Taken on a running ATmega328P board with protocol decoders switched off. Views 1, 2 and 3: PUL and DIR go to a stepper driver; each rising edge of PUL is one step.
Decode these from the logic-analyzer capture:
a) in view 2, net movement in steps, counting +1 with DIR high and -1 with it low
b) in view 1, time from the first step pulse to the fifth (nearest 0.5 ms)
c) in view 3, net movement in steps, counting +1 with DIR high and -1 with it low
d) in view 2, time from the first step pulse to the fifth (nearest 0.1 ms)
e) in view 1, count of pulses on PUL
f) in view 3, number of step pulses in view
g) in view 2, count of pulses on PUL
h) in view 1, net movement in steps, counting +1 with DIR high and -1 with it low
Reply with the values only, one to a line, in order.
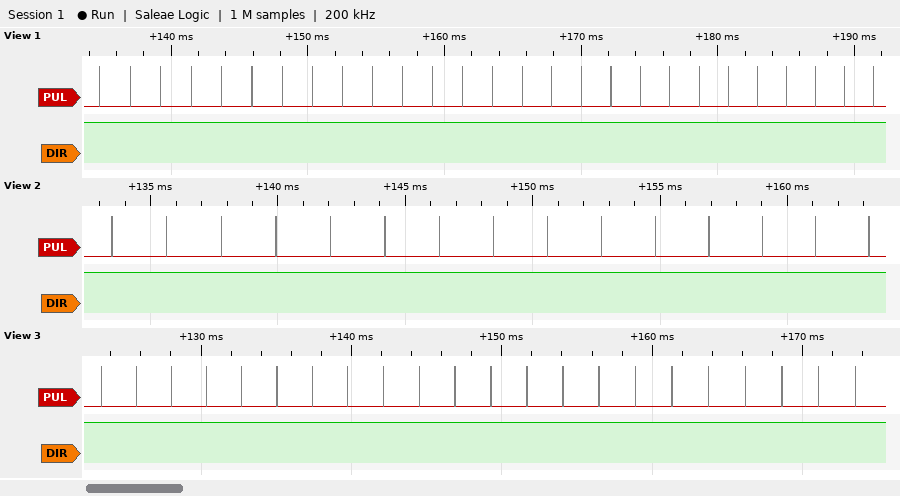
+15
9.0 ms
+22
8.6 ms
27
22
15
+27
